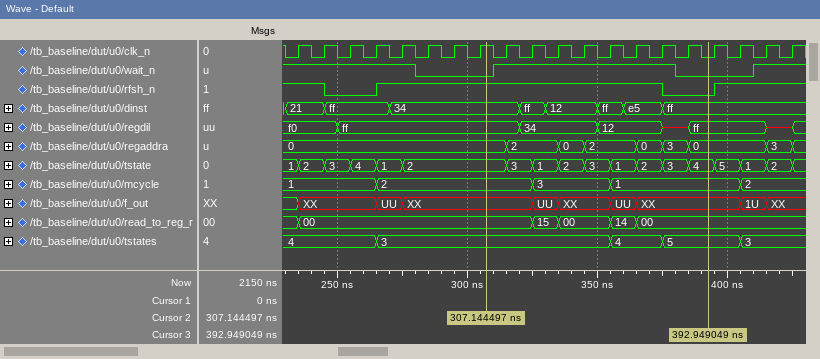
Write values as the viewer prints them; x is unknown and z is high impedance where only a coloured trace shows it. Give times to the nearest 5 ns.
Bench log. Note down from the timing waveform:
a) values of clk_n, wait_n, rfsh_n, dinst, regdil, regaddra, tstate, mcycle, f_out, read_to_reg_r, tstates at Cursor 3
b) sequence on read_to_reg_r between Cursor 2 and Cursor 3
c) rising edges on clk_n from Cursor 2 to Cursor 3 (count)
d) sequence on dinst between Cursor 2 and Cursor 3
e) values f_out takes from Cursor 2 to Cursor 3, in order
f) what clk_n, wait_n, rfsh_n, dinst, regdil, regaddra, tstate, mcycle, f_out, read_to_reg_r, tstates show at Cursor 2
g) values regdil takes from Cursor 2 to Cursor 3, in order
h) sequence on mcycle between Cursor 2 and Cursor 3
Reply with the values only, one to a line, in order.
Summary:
clk_n=0, wait_n=0, rfsh_n=0, dinst=ff, regdil=ff, regaddra=0, tstate=4, mcycle=1, f_out=XX, read_to_reg_r=00, tstates=5
00, 15, 00, 14, 00
8
34, ff, 12, ff, e5, ff
XX, UU, XX, UU, XX
clk_n=1, wait_n=0, rfsh_n=1, dinst=34, regdil=ff, regaddra=0, tstate=2, mcycle=2, f_out=XX, read_to_reg_r=00, tstates=3
ff, 34, 12, x, ff
2, 3, 1
